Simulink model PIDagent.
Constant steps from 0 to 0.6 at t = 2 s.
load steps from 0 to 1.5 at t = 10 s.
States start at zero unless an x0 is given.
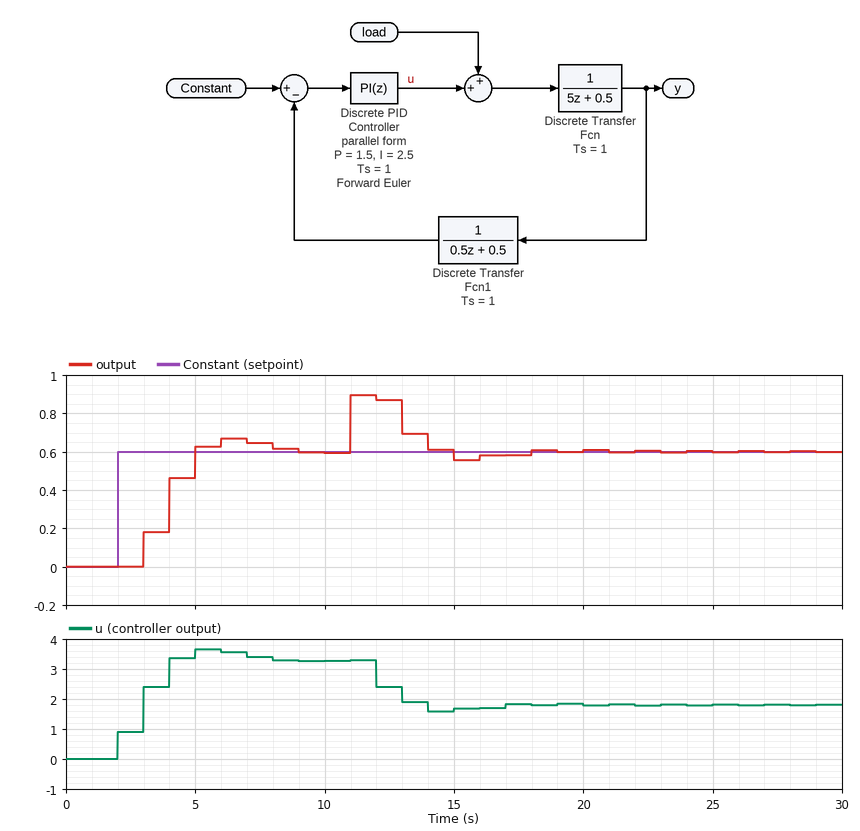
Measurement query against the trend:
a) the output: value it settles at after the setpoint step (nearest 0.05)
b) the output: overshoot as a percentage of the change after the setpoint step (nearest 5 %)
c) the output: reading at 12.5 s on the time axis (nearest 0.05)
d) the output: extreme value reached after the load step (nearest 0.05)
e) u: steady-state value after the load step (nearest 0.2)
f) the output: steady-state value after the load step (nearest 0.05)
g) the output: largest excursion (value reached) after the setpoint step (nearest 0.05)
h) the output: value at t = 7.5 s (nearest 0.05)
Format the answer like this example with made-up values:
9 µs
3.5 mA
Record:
0.60
10 %
0.85
0.90
1.8
0.60
0.65
0.65
